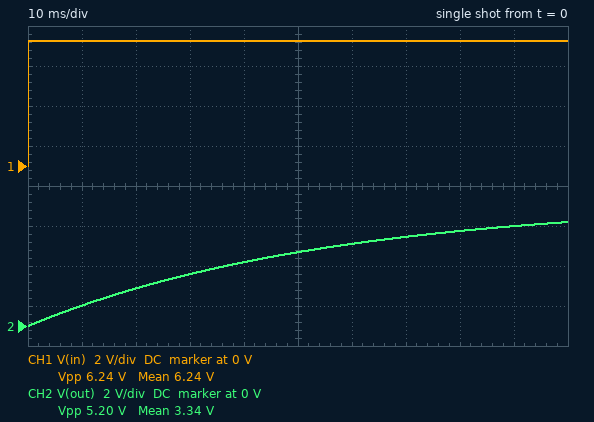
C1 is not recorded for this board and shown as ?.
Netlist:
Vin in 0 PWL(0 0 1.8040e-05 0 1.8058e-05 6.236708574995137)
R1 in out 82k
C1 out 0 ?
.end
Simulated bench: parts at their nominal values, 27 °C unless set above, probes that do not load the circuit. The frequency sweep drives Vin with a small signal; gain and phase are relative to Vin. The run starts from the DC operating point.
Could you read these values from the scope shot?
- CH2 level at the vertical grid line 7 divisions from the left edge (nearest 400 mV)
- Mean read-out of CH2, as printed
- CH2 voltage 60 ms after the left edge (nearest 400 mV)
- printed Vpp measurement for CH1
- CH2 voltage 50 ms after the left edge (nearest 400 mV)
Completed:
4.4 V
3.34 V
4.0 V
6.24 V
3.6 V
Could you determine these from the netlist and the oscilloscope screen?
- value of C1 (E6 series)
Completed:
680 nF
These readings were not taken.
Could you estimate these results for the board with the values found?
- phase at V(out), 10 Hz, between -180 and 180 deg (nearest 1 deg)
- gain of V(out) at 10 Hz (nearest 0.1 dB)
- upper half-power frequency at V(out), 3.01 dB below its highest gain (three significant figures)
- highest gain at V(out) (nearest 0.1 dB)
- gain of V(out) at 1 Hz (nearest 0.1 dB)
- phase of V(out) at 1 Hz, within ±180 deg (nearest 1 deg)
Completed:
-74 deg
-11.2 dB
2.85 Hz
0 dB
-0.5 dB
-19 deg
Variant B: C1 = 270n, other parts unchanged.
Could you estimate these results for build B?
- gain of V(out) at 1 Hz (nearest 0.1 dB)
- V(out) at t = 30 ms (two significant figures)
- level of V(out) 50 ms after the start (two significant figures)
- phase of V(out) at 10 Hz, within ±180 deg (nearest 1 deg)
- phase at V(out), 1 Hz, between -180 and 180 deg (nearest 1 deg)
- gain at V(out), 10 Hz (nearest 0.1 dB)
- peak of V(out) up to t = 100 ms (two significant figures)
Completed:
-0.1 dB
4.6 V
5.6 V
-54 deg
-8 deg
-4.7 dB
6.2 V
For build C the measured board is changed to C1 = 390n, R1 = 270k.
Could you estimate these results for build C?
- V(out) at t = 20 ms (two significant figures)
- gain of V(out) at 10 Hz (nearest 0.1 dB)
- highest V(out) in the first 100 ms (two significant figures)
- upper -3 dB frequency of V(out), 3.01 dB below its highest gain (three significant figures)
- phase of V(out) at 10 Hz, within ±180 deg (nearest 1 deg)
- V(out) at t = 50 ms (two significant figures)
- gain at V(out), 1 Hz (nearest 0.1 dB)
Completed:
1.1 V
-16.5 dB
3.8 V
1.51 Hz
-81 deg
2.4 V
-1.6 dB
